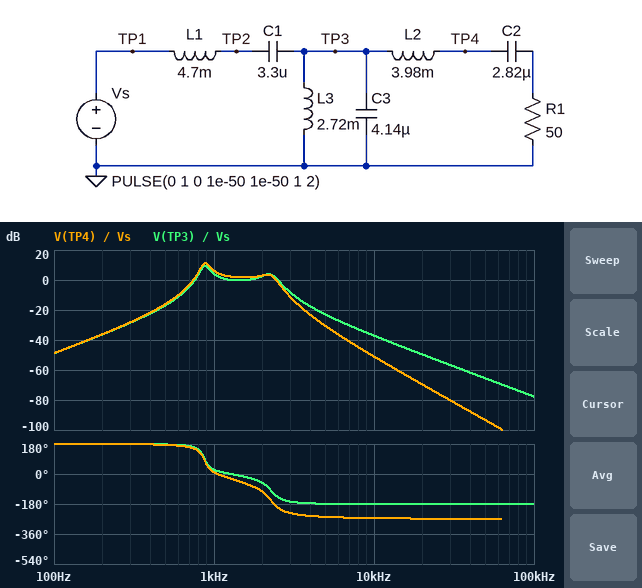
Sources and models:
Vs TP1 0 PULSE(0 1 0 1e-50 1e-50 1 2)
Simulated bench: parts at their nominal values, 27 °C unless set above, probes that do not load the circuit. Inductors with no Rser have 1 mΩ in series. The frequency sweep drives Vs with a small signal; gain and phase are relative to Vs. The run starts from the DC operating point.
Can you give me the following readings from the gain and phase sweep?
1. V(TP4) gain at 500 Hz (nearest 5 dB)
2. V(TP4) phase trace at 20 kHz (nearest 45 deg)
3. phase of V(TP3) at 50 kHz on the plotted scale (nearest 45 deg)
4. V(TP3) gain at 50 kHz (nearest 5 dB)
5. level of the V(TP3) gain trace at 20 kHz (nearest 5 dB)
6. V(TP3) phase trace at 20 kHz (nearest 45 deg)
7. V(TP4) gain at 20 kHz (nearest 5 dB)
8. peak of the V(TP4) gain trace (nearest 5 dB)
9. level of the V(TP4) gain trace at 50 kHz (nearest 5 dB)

-15 dB
-270 deg
-180 deg
-65 dB
-50 dB
-180 deg
-70 dB
10 dB
-95 dB
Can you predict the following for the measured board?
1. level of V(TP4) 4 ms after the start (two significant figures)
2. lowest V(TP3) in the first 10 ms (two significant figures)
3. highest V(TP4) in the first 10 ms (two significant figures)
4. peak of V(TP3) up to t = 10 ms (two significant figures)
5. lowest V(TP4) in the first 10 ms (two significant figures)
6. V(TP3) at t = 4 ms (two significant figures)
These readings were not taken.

-120 mV
-480 mV
420 mV
410 mV
-580 mV
-93 mV
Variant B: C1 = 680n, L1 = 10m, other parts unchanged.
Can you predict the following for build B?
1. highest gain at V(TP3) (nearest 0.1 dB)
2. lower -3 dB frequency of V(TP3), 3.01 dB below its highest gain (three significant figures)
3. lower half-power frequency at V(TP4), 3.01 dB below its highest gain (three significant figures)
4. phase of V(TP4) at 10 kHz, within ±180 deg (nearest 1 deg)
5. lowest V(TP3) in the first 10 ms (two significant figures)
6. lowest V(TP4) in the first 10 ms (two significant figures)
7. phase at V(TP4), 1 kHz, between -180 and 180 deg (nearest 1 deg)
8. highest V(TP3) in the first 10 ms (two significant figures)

5.2 dB
2.06 kHz
2.02 kHz
95 deg
-270 mV
-290 mV
125 deg
210 mV
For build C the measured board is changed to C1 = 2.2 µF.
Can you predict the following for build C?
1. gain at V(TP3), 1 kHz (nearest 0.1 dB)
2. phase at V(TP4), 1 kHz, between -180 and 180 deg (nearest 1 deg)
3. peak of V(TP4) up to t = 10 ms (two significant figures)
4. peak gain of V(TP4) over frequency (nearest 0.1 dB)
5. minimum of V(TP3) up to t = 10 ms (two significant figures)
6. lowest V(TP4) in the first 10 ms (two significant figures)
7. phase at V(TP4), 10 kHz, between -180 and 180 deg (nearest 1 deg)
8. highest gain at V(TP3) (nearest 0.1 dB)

4.2 dB
74 deg
360 mV
6.4 dB
-490 mV
-560 mV
95 deg
5.8 dB
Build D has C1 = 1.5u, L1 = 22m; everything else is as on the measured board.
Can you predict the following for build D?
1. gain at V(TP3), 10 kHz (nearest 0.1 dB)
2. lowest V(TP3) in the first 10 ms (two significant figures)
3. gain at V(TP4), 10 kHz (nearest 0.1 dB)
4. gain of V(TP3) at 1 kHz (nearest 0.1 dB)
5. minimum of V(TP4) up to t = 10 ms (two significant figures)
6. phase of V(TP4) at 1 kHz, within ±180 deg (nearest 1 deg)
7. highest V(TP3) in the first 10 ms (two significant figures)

-50.7 dB
-180 mV
-64.6 dB
-5.2 dB
-230 mV
-31 deg
150 mV
